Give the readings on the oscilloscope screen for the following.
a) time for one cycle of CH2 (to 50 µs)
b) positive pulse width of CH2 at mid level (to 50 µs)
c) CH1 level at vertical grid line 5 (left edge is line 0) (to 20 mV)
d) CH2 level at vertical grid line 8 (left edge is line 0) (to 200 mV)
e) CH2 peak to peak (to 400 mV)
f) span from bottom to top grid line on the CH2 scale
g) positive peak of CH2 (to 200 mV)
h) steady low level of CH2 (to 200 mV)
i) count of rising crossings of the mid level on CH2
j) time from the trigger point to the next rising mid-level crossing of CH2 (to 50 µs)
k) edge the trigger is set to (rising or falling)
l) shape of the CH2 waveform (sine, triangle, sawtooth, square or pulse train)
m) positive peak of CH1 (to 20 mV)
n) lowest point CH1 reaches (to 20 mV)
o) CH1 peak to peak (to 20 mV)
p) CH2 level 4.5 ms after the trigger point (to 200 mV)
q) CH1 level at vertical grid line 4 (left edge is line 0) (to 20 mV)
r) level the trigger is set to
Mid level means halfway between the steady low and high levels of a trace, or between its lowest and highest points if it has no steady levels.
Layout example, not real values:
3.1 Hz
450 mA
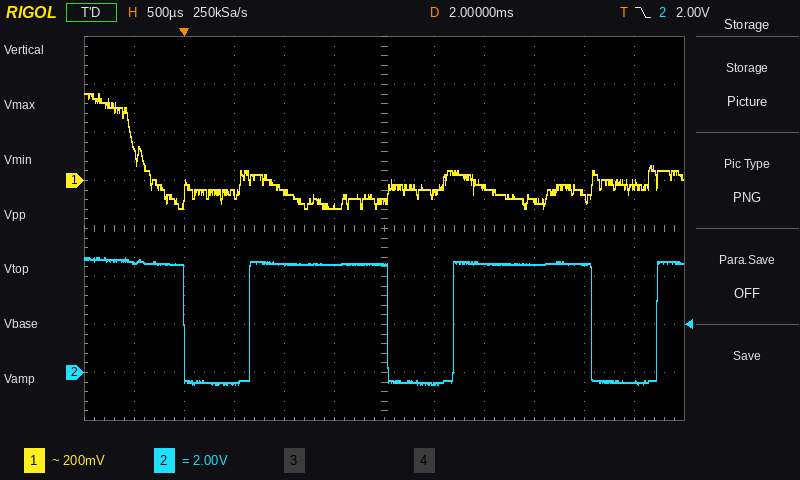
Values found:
2.05 ms
1.40 ms
-100 mV
4.6 V
5.2 V
16 V
4.8 V
-400 mV
3
650 µs
falling
pulse train
360 mV
-120 mV
480 mV
-400 mV
-40 mV
2.00 V
